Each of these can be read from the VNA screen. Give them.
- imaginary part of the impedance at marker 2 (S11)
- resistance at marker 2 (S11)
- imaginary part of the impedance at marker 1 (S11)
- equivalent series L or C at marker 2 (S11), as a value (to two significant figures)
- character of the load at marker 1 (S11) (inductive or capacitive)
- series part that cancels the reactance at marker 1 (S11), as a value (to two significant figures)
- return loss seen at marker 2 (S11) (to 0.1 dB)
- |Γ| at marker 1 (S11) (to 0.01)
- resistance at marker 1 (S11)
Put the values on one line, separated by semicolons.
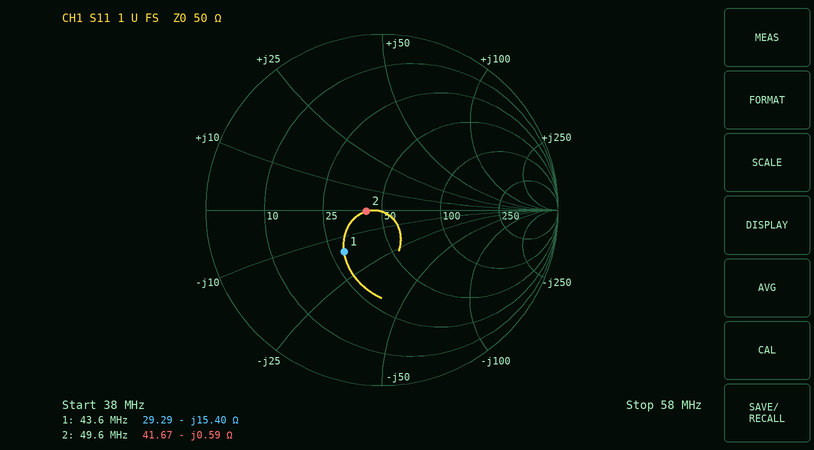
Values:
-0.59 Ω; 41.67 Ω; -15.40 Ω; 5.4 nF; capacitive; 56 nH; 20.8 dB; 0.32; 29.29 Ω
